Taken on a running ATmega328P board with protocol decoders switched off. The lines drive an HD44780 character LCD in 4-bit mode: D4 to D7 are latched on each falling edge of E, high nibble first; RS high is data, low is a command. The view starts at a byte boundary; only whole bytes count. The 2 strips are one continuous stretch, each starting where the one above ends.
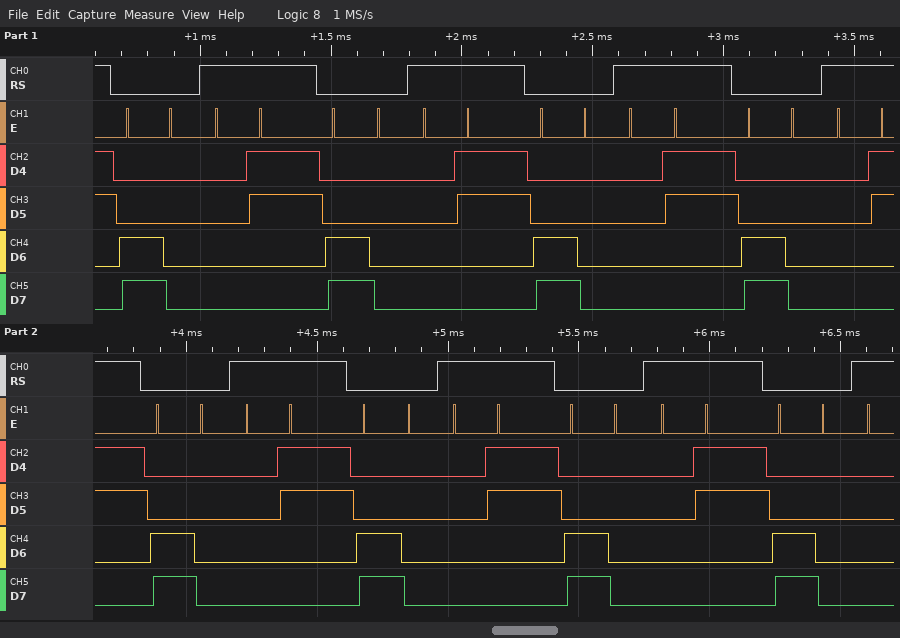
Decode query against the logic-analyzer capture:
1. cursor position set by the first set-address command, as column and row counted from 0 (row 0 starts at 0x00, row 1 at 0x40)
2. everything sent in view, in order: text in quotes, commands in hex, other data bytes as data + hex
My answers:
column 0, row 1
0xC0 data 03 0xC0 data 03 0xC0 data 03 0xC0 data 03 0xC0 data 03 0xC0 data 03 0xC0 data 03 0xC0
